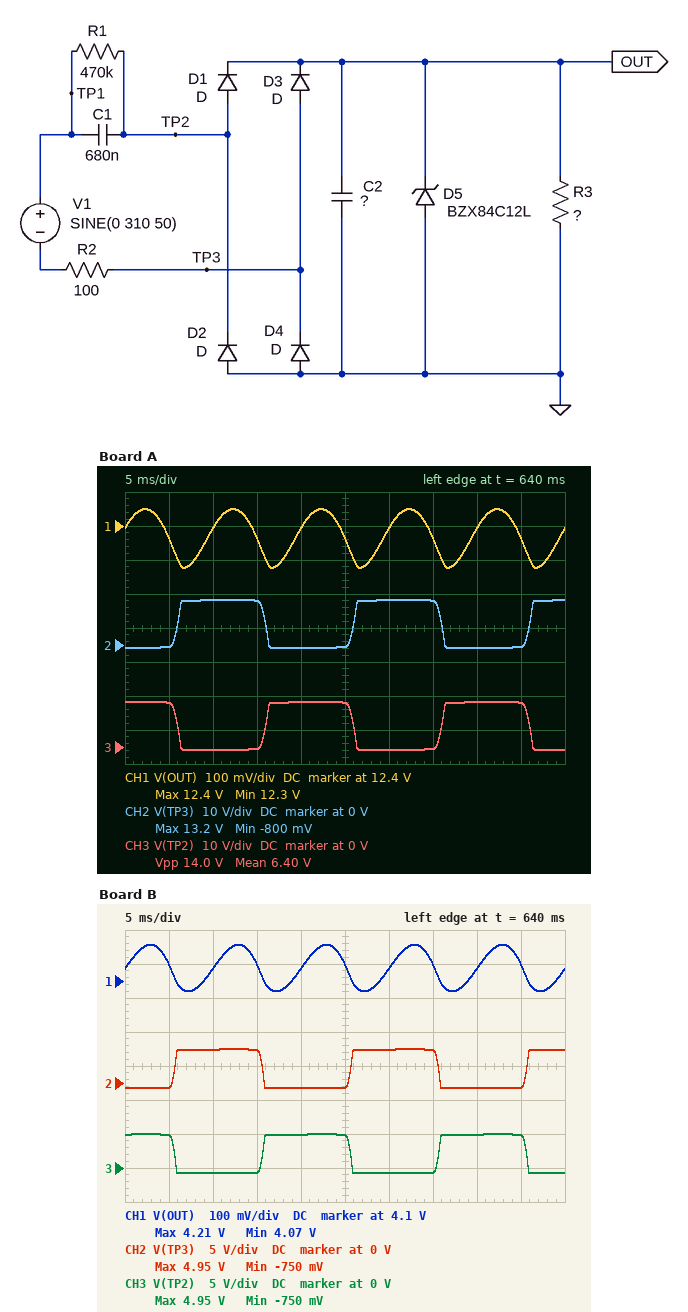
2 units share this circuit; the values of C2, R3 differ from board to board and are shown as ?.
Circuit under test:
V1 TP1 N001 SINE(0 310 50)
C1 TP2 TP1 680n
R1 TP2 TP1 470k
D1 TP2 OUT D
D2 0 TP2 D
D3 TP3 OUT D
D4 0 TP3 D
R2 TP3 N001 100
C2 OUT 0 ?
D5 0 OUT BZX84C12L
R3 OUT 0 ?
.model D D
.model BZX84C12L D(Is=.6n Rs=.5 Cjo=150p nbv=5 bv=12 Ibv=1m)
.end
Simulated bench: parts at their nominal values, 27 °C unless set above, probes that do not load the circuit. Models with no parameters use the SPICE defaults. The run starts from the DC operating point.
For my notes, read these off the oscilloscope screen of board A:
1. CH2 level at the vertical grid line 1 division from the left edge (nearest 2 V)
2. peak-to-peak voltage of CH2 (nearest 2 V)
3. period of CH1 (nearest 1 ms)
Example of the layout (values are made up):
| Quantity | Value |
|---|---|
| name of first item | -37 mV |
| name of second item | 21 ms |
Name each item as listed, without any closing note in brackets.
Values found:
| Quantity | Value |
|---|---|
| CH2 level at the vertical grid line 1 division from the left edge | 0 V |
| peak-to-peak voltage of CH2 | 14 V |
| period of CH1 | 10 ms |
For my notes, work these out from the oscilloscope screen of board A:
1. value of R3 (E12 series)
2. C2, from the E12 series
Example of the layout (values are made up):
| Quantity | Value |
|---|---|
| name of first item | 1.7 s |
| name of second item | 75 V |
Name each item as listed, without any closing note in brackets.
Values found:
| Quantity | Value |
|---|---|
| value of R3 | 560 Ω |
| C2, from the E12 series | 560 µF |
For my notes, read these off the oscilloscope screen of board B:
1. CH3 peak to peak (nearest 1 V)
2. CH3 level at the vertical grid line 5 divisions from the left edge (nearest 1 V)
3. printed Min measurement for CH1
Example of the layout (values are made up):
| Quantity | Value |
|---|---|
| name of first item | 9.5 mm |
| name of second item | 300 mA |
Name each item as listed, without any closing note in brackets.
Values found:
| Quantity | Value |
|---|---|
| CH3 peak to peak | 6 V |
| CH3 level at the vertical grid line 5 divisions from the left edge | 5 V |
| printed Min measurement for CH1 | 4.07 V |
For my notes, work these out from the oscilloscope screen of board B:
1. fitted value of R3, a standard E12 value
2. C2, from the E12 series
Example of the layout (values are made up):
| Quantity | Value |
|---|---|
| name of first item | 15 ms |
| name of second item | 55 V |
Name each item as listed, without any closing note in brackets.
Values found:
| Quantity | Value |
|---|---|
| fitted value of R3, a standard E12 value | 100 Ω |
| C2, from the E12 series | 680 µF |
